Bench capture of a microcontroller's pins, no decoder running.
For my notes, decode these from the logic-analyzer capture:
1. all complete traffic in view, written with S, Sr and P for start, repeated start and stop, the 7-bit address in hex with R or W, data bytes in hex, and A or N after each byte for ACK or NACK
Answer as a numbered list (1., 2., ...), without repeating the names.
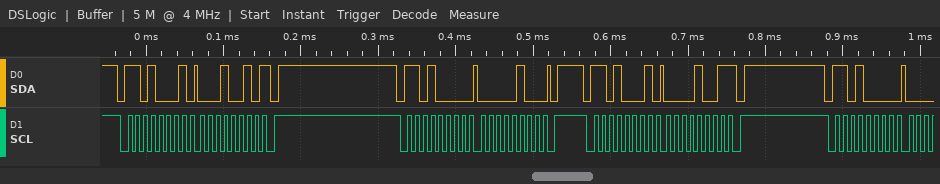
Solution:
1. S 68R A 12 N P S 68W A 04 A P S 68R A 09 N P S 68W A
